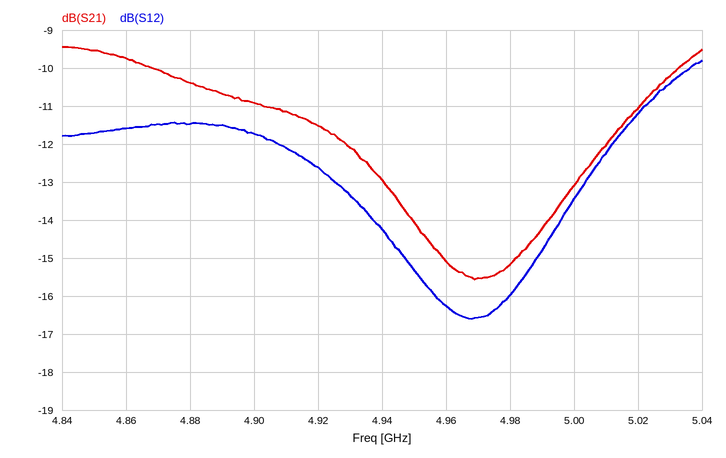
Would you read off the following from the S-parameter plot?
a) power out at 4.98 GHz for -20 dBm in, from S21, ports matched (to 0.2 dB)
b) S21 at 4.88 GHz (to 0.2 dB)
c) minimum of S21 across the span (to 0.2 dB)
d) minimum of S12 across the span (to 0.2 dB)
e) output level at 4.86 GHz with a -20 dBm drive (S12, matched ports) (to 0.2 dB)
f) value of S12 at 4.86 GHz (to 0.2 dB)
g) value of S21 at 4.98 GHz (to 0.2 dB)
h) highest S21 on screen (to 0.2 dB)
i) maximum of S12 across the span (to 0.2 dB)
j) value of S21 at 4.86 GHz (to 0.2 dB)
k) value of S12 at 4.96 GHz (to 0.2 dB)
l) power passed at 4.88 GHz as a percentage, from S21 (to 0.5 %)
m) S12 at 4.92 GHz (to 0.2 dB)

-35.2 dBm
-10.4 dB
-15.6 dB
-16.6 dB
-31.6 dBm
-11.6 dB
-15.2 dB
-9.4 dB
-9.8 dB
-9.8 dB
-16.2 dB
9.0 %
-12.6 dB
